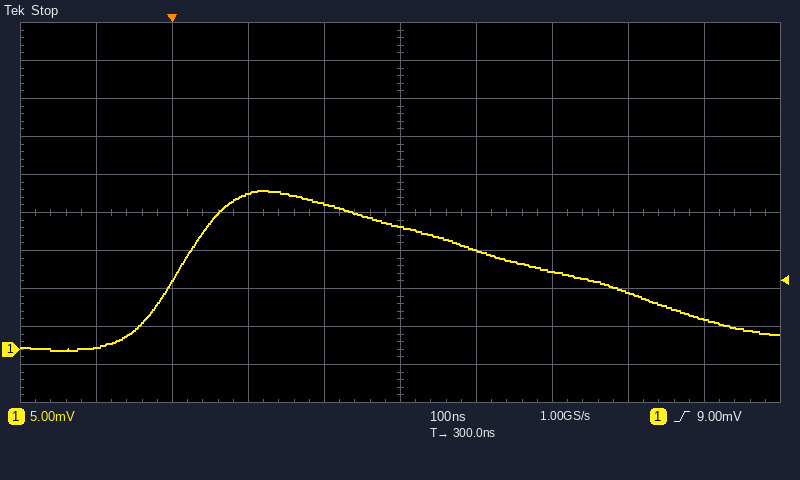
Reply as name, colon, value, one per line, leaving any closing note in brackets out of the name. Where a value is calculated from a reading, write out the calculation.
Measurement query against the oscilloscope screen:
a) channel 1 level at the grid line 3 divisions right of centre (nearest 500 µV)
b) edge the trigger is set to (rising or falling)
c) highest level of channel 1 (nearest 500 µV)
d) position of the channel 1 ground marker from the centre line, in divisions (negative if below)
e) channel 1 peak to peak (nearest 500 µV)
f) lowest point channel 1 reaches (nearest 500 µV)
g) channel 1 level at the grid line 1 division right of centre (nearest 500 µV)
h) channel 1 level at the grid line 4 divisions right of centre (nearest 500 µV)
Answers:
channel 1 level at the grid line 3 divisions right of centre: 7.5 mV
edge the trigger is set to: rising
highest level of channel 1: 21.0 mV
position of the channel 1 ground marker from the centre line, in divisions: -3.6 div
channel 1 peak to peak: 21.0 mV − (0.0 mV) = 21.0 mV
lowest point channel 1 reaches: 0.0 mV
channel 1 level at the grid line 1 division right of centre: 13.0 mV
channel 1 level at the grid line 4 divisions right of centre: 4.0 mV
